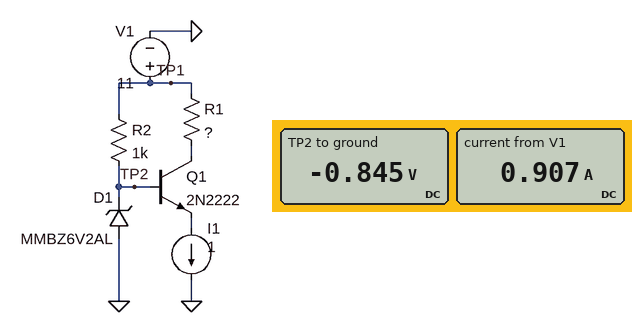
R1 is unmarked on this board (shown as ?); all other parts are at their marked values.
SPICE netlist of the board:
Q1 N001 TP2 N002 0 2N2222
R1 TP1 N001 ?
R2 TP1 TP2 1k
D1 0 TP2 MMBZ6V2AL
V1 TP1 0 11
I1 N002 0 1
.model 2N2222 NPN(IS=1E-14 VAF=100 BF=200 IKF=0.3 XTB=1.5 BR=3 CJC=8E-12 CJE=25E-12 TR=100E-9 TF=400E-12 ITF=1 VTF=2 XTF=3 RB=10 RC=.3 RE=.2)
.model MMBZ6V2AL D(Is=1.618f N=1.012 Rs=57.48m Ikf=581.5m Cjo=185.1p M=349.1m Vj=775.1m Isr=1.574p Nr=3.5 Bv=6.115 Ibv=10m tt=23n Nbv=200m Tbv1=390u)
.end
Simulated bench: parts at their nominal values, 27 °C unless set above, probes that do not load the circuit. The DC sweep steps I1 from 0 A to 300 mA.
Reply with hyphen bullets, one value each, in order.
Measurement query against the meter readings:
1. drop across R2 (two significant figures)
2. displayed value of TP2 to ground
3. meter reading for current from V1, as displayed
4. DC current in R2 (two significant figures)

- 12 V
- -0.845 V
- 0.907 A
- 12 mA
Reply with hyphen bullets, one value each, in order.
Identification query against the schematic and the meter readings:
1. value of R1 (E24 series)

- 15 Ω
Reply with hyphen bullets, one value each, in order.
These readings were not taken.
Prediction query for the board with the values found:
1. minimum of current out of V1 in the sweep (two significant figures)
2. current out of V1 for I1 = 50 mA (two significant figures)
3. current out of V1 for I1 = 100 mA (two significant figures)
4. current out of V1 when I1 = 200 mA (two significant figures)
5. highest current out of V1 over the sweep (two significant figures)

- 4.9 mA
- 55 mA
- 100 mA
- 200 mA
- 300 mA
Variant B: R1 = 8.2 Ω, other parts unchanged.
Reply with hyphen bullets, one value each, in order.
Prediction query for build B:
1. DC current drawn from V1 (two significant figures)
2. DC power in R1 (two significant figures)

- 990 mA
- 7.9 W
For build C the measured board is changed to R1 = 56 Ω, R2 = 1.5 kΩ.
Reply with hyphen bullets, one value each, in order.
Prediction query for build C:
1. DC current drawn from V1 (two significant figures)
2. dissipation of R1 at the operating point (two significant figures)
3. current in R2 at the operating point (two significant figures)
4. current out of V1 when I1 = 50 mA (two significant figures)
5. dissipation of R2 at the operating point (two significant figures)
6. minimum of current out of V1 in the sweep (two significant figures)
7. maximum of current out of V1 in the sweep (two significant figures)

- 350 mA
- 6.6 W
- 8.0 mA
- 53 mA
- 95 mW
- 3.3 mA
- 240 mA
